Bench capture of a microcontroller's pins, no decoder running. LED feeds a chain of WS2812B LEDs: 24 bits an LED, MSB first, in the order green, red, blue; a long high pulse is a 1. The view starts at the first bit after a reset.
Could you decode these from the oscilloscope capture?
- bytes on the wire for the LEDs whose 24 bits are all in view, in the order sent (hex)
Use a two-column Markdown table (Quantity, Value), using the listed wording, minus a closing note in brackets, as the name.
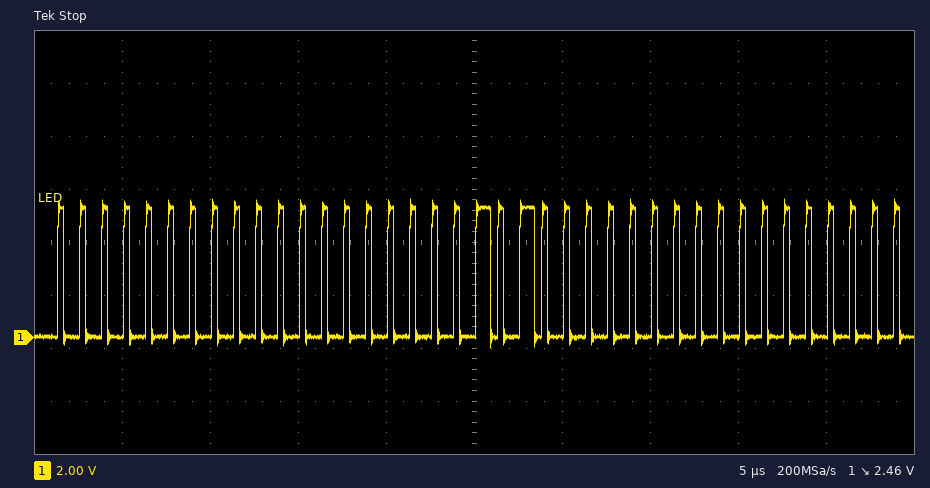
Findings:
| Quantity | Value |
|---|---|
| bytes on the wire for the LEDs whose 24 bits are all in view, in the order sent | 00 00 14 |
